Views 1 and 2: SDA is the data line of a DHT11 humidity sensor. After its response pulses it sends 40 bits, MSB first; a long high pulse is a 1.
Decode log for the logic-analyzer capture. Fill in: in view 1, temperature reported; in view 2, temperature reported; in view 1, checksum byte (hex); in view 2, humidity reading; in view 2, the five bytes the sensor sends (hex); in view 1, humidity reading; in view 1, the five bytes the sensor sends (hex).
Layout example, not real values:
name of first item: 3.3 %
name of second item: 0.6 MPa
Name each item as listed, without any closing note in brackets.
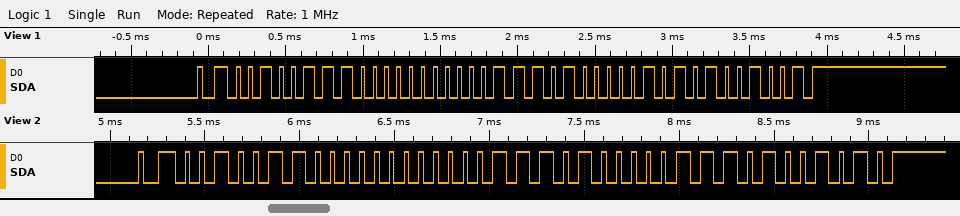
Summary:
in view 1, temperature reported: 29.5 °C
in view 2, temperature reported: 29.7 °C
in view 1, checksum byte: 0x49
in view 2, humidity reading: 38 %
in view 2, the five bytes the sensor sends: 26 00 1D 07 4A
in view 1, humidity reading: 39 %
in view 1, the five bytes the sensor sends: 27 00 1D 05 49
